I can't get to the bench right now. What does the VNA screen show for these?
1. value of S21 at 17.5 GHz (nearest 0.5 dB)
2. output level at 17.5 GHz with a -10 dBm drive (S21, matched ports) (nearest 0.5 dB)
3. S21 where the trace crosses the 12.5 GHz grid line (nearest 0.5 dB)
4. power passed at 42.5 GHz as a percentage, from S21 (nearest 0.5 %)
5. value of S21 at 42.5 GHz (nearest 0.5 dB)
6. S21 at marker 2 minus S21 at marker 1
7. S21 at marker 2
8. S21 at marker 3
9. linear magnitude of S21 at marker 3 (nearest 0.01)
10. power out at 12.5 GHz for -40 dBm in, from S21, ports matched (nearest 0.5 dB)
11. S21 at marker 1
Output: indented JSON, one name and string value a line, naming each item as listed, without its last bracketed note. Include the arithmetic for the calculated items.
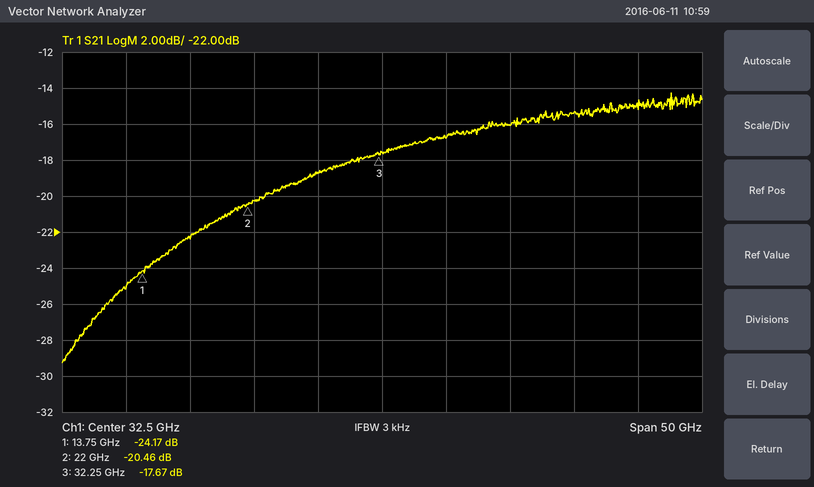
{
  "value of S21 at 17.5 GHz": "-22.5 dB",
  "output level at 17.5 GHz with a -10 dBm drive (S21, matched ports)": "-10 dBm + (-22.5 dB) = -32.5 dBm",
  "S21 where the trace crosses the 12.5 GHz grid line": "-25.0 dB",
  "power passed at 42.5 GHz as a percentage, from S21": "10^(-16/10) ≈ 2.5 %",
  "value of S21 at 42.5 GHz": "-16.0 dB",
  "S21 at marker 2 minus S21 at marker 1": "-20.46 − (-24.17) = 3.71 dB",
  "S21 at marker 2": "-20.46 dB",
  "S21 at marker 3": "-17.67 dB",
  "linear magnitude of S21 at marker 3": "10^(-17.67/20) ≈ 0.13",
  "power out at 12.5 GHz for -40 dBm in, from S21, ports matched": "-40 dBm + (-25.0 dB) = -65.0 dBm",
  "S21 at marker 1": "-24.17 dB"
}
